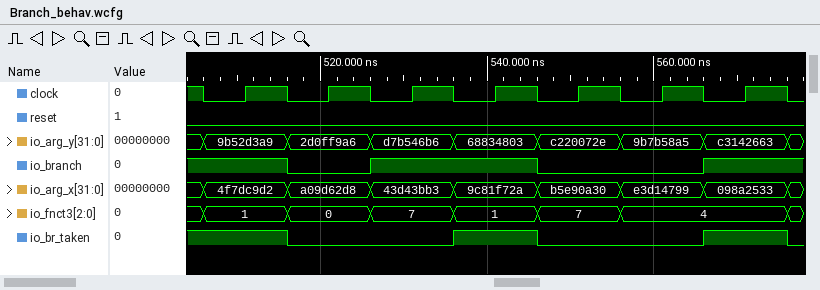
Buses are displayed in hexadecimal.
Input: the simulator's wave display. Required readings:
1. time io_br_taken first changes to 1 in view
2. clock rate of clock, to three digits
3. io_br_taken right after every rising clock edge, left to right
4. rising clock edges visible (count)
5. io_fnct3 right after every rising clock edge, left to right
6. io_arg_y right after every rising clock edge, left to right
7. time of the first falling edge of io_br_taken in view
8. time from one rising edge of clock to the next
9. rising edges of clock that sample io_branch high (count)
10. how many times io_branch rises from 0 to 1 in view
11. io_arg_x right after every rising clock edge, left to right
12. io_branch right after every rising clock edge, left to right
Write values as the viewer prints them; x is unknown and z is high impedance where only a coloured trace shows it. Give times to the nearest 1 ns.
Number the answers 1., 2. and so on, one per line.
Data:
1. 536 ns
2. 100 MHz
3. 1 0 0 1 0 0 1
4. 7
5. 1, 0, 7, 1, 7, 4, 4
6. 9b52d3a9, 2d0ff9a6, d7b546b6, 68834803, c220072e, 9b7b58a5, c3142663
7. 516 ns
8. 10 ns
9. 4
10. 2
11. 4f7dc9d2, a09d62d8, 43d43bb3, 9c81f72a, b5e90a30, e3d14799, 098a2533
12. 1 0 1 1 0 0 1
